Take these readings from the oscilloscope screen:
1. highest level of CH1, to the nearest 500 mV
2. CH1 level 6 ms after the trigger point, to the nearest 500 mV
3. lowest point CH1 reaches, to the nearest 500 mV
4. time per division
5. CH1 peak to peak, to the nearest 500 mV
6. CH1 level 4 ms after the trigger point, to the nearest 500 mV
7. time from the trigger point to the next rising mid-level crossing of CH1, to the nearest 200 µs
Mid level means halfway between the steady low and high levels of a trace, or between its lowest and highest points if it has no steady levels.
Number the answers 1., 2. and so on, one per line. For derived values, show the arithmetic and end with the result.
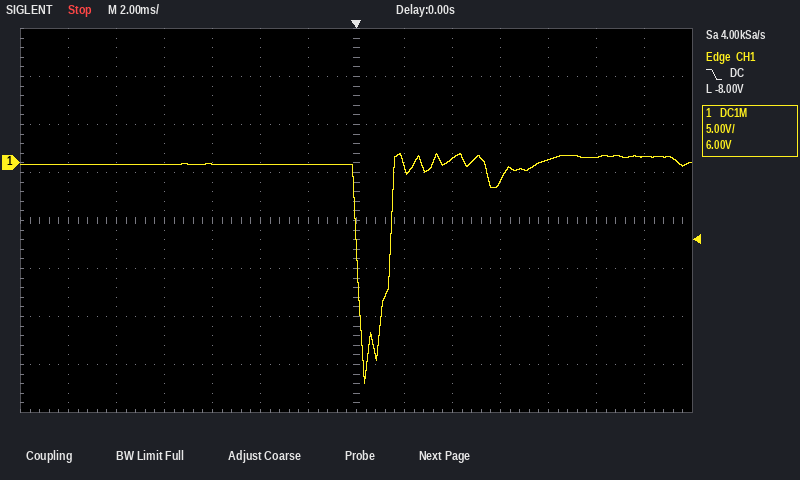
1. 1.0 V
2. -2.0 V
3. -23.0 V
4. 2 ms
5. 1.0 V − (-23.0 V) = 24.0 V
6. 500 mV
7. 1.4 ms
